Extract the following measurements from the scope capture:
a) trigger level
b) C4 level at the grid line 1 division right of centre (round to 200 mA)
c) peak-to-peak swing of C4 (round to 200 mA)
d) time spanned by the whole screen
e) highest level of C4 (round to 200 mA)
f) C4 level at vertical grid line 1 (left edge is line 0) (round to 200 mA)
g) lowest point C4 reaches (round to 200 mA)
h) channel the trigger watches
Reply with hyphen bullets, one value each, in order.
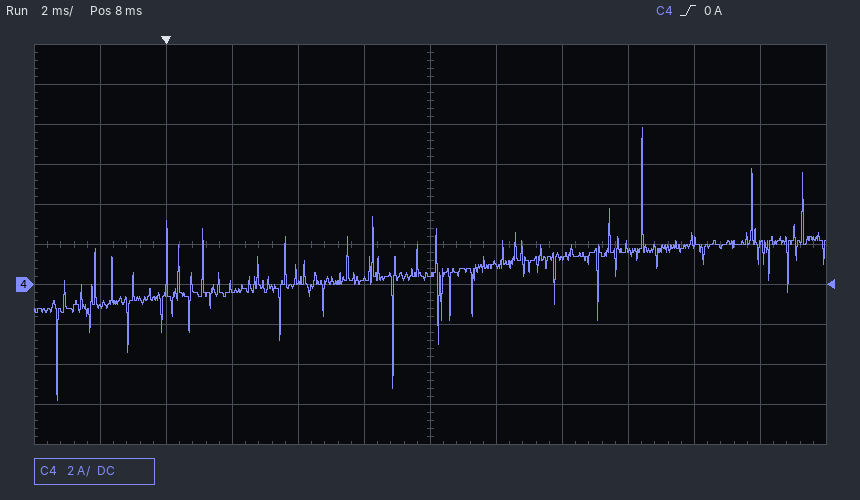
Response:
- 0 A
- 1.0 A
- 13.6 A
- 24 ms
- 7.8 A
- -1.0 A
- -5.8 A
- C4
